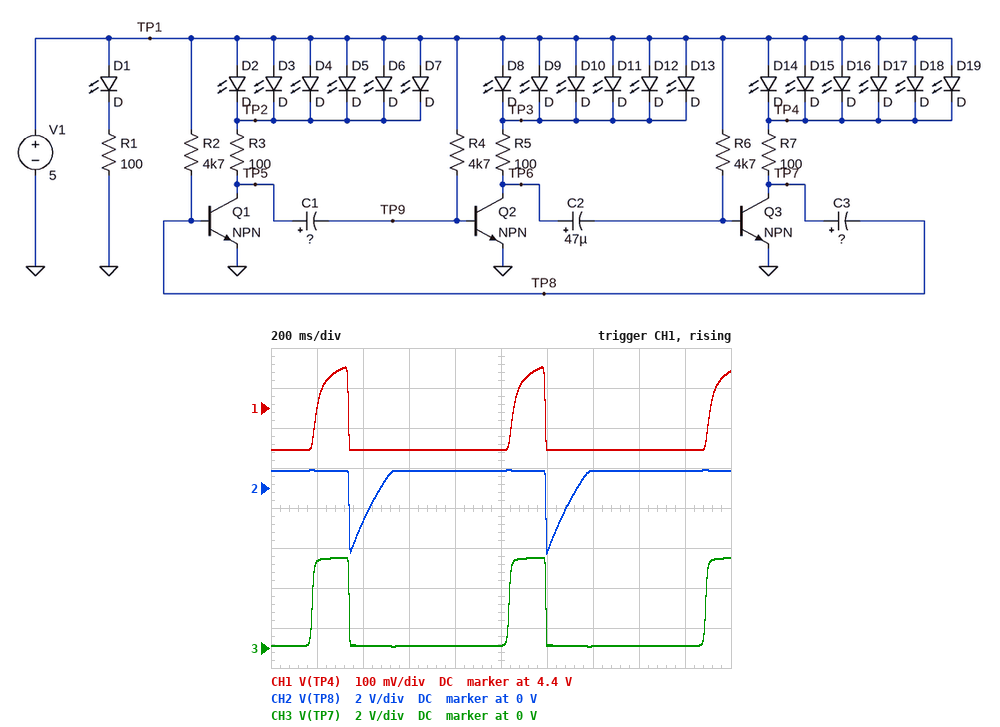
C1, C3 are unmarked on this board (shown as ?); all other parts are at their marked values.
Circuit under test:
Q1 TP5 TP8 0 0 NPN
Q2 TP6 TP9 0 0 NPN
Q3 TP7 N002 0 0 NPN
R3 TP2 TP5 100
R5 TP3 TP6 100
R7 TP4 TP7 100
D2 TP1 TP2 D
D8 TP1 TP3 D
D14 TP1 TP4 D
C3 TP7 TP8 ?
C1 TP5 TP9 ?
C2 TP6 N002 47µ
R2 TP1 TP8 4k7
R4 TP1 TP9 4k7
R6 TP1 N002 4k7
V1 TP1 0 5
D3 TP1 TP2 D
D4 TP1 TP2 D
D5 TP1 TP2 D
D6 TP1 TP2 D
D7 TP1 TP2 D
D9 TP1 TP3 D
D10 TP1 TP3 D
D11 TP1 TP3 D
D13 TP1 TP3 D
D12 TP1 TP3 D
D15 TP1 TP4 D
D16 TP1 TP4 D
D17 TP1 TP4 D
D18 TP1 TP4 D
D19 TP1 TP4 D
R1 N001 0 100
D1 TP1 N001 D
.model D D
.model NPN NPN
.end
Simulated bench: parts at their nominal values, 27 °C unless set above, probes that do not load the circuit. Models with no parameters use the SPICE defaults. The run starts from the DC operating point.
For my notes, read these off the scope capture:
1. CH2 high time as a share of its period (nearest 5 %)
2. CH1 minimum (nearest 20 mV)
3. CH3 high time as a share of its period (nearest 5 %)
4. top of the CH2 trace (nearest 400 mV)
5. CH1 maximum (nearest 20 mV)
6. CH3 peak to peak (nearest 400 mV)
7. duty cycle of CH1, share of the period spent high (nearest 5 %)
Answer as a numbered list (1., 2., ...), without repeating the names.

1. 90 %
2. 4.30 V
3. 20 %
4. 800 mV
5. 4.50 V
6. 4.4 V
7. 15 %
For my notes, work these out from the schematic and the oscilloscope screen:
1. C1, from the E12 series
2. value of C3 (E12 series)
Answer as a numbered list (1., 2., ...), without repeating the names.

1. 150 µF
2. 56 µF
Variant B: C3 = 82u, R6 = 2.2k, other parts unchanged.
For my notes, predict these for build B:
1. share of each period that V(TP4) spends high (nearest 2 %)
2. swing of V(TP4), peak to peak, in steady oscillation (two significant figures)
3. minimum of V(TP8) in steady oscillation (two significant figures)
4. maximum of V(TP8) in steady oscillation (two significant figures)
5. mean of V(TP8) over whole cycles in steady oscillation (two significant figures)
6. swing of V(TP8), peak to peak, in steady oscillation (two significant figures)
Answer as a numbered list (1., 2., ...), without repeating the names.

1. 6 %
2. 150 mV
3. -3.4 V
4. 890 mV
5. 260 mV
6. 4.3 V
